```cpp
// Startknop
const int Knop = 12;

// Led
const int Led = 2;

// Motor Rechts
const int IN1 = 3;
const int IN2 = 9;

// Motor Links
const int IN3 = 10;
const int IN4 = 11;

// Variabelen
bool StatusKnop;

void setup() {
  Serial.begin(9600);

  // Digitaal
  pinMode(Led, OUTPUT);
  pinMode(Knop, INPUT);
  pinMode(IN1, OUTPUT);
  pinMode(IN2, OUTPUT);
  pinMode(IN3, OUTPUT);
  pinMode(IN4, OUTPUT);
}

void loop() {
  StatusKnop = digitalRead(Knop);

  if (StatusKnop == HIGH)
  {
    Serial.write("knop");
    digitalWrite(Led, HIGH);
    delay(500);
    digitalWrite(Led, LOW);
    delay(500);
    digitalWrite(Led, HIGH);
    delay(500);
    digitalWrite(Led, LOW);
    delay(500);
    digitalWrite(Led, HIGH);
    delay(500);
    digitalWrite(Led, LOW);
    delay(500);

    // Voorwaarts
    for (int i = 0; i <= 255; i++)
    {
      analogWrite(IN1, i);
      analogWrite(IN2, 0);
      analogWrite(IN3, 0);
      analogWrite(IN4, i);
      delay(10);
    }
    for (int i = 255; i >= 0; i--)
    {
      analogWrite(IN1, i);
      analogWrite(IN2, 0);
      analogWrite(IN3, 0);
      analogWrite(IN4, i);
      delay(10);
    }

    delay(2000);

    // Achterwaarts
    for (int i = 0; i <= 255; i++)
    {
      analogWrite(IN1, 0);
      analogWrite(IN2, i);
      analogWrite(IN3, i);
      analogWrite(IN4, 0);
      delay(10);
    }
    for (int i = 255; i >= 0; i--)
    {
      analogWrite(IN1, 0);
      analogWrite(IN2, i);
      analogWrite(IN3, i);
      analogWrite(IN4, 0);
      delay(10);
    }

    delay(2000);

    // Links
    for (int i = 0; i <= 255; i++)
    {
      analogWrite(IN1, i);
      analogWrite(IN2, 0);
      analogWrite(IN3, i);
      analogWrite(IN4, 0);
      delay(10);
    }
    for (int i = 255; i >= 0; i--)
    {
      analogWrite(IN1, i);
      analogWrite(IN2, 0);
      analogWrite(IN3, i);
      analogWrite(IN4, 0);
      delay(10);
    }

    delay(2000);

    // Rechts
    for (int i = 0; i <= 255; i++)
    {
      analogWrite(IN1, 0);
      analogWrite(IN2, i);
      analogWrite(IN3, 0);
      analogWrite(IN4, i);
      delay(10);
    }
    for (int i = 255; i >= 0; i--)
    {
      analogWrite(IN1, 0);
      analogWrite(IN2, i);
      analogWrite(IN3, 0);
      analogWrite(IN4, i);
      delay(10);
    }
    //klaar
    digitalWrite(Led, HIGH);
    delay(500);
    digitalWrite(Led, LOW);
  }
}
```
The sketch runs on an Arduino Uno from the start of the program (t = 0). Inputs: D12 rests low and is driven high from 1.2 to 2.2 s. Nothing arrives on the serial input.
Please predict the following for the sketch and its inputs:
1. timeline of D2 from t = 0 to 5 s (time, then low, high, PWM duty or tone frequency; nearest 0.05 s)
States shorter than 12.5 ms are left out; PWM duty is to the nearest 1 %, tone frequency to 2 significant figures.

0 s low; 1.2 s high; 1.7 s low; 2.2 s high; 2.7 s low; 3.2 s high; 3.7 s low
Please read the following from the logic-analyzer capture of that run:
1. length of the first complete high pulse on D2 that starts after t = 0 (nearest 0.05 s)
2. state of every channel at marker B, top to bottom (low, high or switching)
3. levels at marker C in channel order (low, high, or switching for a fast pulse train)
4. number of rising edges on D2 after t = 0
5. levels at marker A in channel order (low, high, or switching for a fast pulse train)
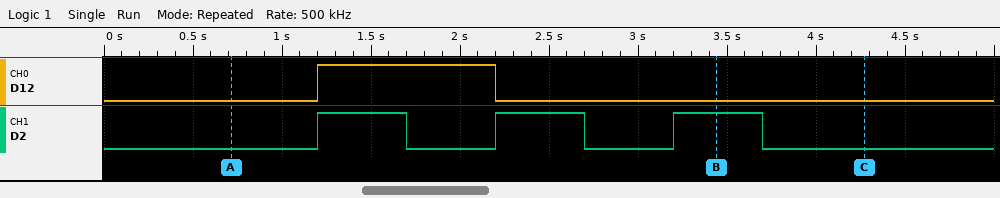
0.50 s
D12 low, D2 high
D12 low, D2 low
3
D12 low, D2 low
